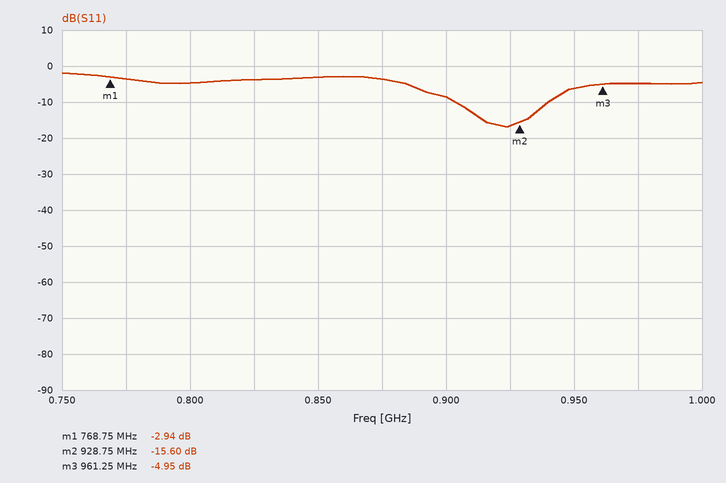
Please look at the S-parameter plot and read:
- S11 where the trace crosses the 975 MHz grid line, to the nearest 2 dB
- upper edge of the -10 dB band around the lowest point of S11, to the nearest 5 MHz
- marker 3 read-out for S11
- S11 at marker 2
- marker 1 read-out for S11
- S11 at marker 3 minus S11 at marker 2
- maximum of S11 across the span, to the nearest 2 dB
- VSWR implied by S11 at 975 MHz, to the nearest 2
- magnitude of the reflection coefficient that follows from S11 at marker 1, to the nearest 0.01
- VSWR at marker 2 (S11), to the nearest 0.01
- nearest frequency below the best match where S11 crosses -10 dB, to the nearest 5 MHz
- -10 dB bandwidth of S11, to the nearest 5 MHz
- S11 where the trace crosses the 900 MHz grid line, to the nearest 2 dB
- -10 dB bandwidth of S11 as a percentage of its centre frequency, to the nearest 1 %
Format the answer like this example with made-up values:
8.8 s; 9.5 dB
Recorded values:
-4 dB; 940 MHz; -4.95 dB; -15.60 dB; -2.94 dB; 10.65 dB; -2 dB; 4; 0.71; 1.40; 905 MHz; 35 MHz; -8 dB; 4 %
